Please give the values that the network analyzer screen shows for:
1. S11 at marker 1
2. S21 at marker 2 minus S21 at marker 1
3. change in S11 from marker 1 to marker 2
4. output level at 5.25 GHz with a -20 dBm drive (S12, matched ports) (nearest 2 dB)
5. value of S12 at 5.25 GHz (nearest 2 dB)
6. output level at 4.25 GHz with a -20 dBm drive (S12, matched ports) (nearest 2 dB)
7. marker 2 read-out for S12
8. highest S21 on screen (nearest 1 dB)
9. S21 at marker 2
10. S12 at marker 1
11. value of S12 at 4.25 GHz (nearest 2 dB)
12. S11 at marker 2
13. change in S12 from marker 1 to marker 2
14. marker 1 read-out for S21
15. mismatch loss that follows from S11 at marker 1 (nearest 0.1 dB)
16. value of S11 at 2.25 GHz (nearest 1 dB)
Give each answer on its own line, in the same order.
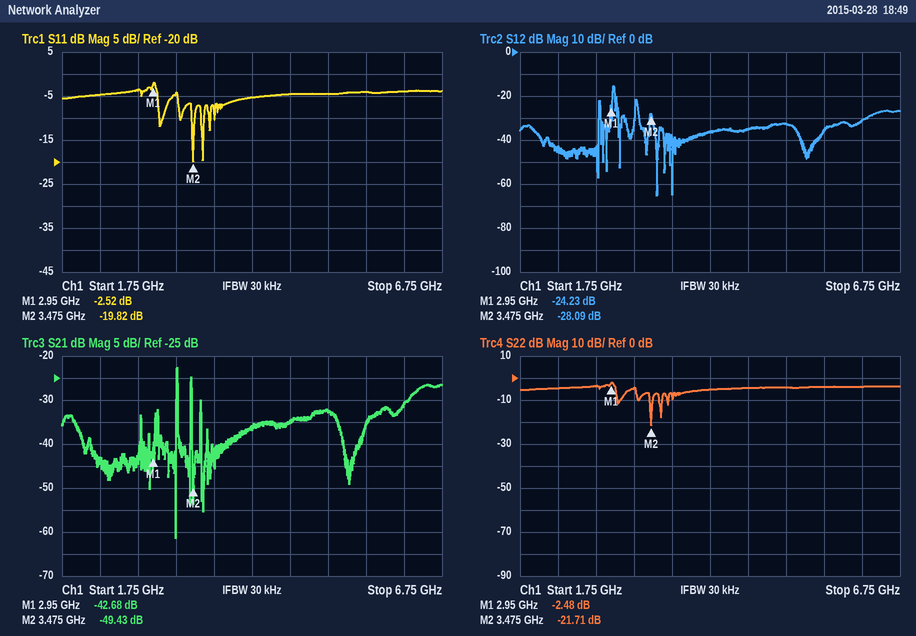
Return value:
-2.52 dB
-6.75 dB
-17.30 dB
-52 dBm
-32 dB
-56 dBm
-28.09 dB
-23 dB
-49.43 dB
-24.23 dB
-36 dB
-19.82 dB
-3.86 dB
-42.68 dB
3.6 dB
-5 dB
